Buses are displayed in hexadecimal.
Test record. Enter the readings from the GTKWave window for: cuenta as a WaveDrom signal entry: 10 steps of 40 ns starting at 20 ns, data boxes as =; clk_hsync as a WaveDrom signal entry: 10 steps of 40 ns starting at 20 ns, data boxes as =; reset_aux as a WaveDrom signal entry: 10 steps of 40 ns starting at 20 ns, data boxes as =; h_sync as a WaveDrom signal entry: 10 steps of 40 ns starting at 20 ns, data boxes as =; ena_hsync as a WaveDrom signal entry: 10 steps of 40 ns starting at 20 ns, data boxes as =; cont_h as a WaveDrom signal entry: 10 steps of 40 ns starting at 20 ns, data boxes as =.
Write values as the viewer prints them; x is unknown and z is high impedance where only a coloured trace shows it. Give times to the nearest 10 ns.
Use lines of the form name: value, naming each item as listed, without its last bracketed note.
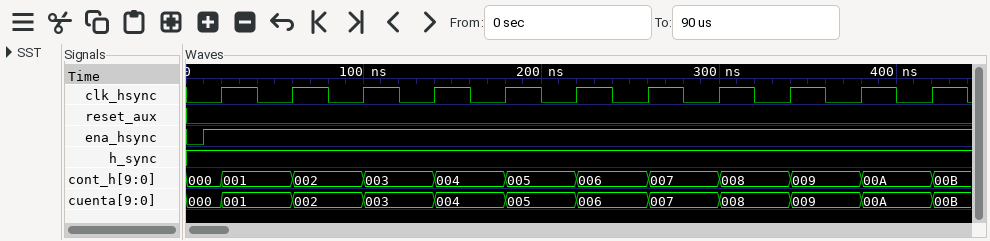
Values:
cuenta as a WaveDrom signal entry: 10 steps of 40 ns starting at 20 ns, data boxes as =: {name: 'cuenta', wave: '==========', data: '001 002 003 004 005 006 007 008 009 00A'}
clk_hsync as a WaveDrom signal entry: 10 steps of 40 ns starting at 20 ns, data boxes as =: {name: 'clk_hsync', wave: 'p.........'}
reset_aux as a WaveDrom signal entry: 10 steps of 40 ns starting at 20 ns, data boxes as =: {name: 'reset_aux', wave: '0.........'}
h_sync as a WaveDrom signal entry: 10 steps of 40 ns starting at 20 ns, data boxes as =: {name: 'h_sync', wave: '1.........'}
ena_hsync as a WaveDrom signal entry: 10 steps of 40 ns starting at 20 ns, data boxes as =: {name: 'ena_hsync', wave: '1.........'}
cont_h as a WaveDrom signal entry: 10 steps of 40 ns starting at 20 ns, data boxes as =: {name: 'cont_h', wave: '==========', data: '001 002 003 004 005 006 007 008 009 00A'}
